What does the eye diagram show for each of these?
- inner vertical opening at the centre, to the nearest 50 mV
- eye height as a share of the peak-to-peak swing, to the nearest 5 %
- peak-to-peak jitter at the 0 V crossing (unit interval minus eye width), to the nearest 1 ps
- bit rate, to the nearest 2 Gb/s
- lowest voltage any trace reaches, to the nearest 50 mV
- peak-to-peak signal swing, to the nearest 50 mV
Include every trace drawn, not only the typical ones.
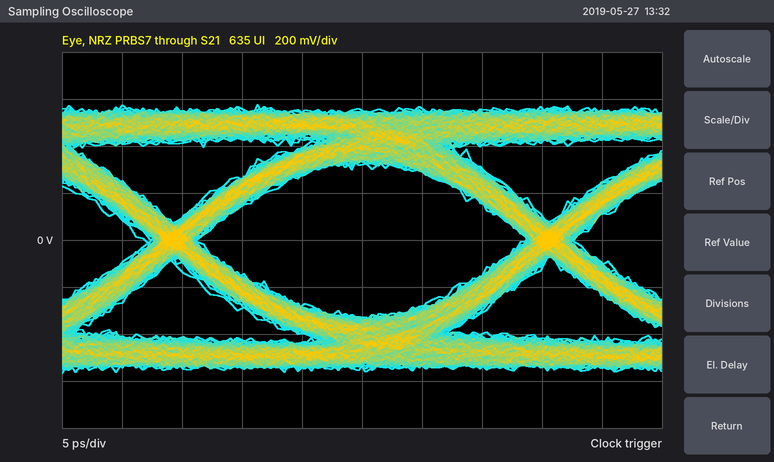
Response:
650 mV
55 %
4 ps
32 Gb/s
-550 mV
1.15 V
